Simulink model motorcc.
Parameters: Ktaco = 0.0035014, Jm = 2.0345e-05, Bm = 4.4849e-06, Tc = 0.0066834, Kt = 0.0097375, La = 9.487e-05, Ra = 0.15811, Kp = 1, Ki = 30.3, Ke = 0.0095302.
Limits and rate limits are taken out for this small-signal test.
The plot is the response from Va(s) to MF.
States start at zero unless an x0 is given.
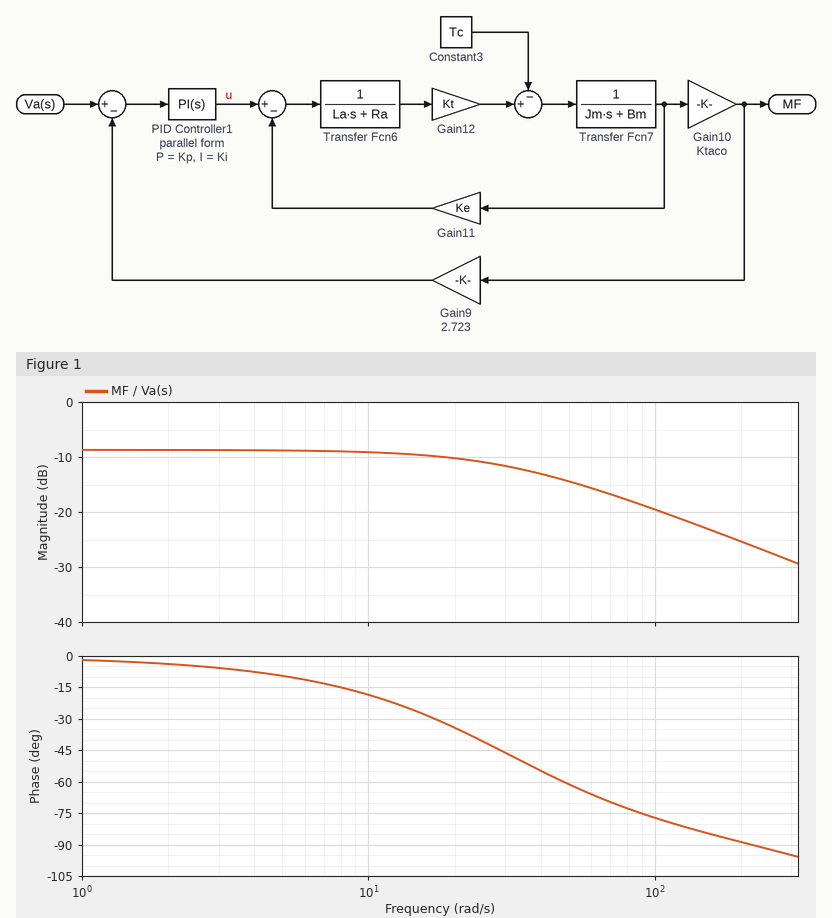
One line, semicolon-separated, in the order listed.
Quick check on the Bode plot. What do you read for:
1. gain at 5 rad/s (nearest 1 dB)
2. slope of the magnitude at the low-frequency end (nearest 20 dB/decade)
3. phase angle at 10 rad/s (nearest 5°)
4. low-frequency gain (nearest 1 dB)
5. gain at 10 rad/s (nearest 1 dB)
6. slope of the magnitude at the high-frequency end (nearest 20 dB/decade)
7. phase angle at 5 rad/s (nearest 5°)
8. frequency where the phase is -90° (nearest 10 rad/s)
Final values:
-9 dB; 0 dB/decade; -20°; -9 dB; -9 dB; -20 dB/decade; -10°; 220 rad/s
